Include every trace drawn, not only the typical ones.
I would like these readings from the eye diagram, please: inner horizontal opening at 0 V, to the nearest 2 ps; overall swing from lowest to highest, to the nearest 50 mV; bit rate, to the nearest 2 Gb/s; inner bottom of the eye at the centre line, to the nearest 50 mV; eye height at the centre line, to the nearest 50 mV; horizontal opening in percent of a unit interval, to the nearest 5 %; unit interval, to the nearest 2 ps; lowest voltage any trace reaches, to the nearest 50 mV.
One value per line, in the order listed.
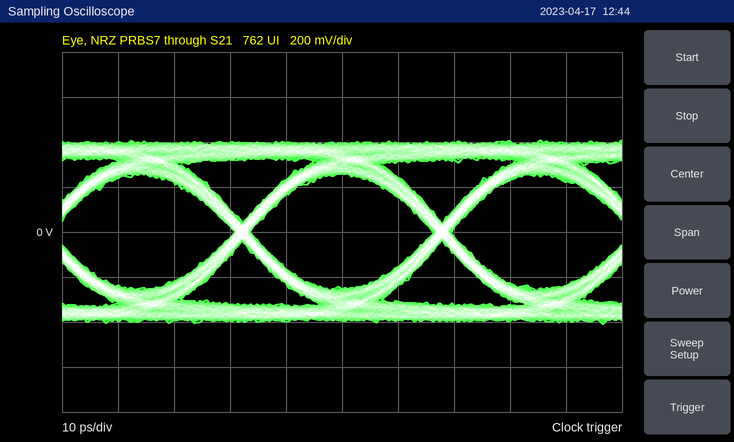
32 ps
800 mV
28 Gb/s
-250 mV
500 mV
90 %
36 ps
-400 mV
